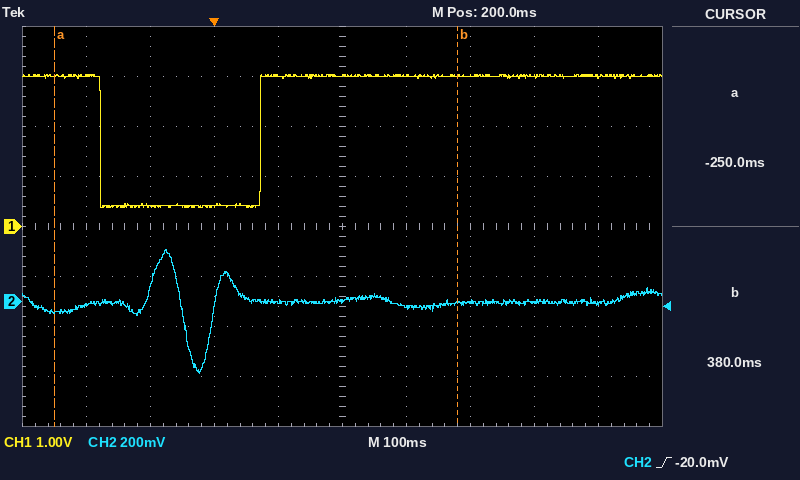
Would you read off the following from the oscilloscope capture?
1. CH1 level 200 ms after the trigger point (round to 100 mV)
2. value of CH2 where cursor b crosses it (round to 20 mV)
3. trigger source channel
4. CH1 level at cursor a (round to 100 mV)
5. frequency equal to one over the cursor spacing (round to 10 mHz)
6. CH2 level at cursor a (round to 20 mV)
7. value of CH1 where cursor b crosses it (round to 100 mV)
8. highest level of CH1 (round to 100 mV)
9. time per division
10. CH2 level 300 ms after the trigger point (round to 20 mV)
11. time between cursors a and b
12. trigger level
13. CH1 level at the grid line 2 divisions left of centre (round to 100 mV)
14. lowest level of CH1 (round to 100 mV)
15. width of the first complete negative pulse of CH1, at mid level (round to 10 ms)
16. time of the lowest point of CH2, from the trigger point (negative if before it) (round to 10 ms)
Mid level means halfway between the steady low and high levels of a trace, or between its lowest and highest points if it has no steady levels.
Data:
3.0 V
0 mV
CH2
3.0 V
1.59 Hz
-40 mV
3.0 V
3.0 V
100 ms
-20 mV
630 ms
-20.0 mV
400 mV
400 mV
250 ms
-20 ms
